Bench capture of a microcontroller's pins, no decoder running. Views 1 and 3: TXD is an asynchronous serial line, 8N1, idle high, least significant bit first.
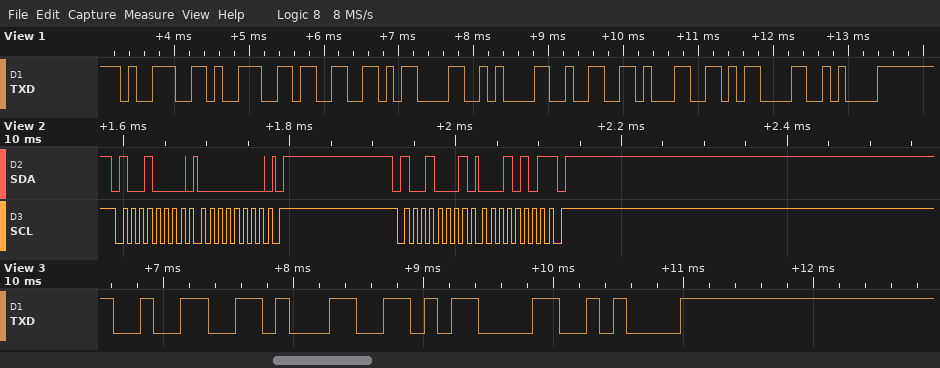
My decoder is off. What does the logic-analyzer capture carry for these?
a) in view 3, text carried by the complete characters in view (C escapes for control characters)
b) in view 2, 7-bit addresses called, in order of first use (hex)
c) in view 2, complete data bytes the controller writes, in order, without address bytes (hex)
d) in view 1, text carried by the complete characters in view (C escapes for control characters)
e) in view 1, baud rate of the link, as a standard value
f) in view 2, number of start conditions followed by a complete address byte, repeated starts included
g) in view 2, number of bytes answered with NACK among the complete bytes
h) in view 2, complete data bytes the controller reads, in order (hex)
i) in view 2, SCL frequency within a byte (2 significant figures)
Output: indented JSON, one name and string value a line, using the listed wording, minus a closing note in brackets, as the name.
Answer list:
{
  "in view 3, text carried by the complete characters in view": "\"21\\r\\n\"",
  "in view 2, 7-bit addresses called, in order of first use": "0x48",
  "in view 2, complete data bytes the controller writes, in order, without address bytes": "00",
  "in view 1, text carried by the complete characters in view": "\"993\\r\\n21\\r\\n\"",
  "in view 1, baud rate of the link, as a standard value": "9600 baud",
  "in view 2, number of start conditions followed by a complete address byte, repeated starts included": "2",
  "in view 2, number of bytes answered with NACK among the complete bytes": "1",
  "in view 2, complete data bytes the controller reads, in order": "15",
  "in view 2, SCL frequency within a byte": "100 kHz"
}
